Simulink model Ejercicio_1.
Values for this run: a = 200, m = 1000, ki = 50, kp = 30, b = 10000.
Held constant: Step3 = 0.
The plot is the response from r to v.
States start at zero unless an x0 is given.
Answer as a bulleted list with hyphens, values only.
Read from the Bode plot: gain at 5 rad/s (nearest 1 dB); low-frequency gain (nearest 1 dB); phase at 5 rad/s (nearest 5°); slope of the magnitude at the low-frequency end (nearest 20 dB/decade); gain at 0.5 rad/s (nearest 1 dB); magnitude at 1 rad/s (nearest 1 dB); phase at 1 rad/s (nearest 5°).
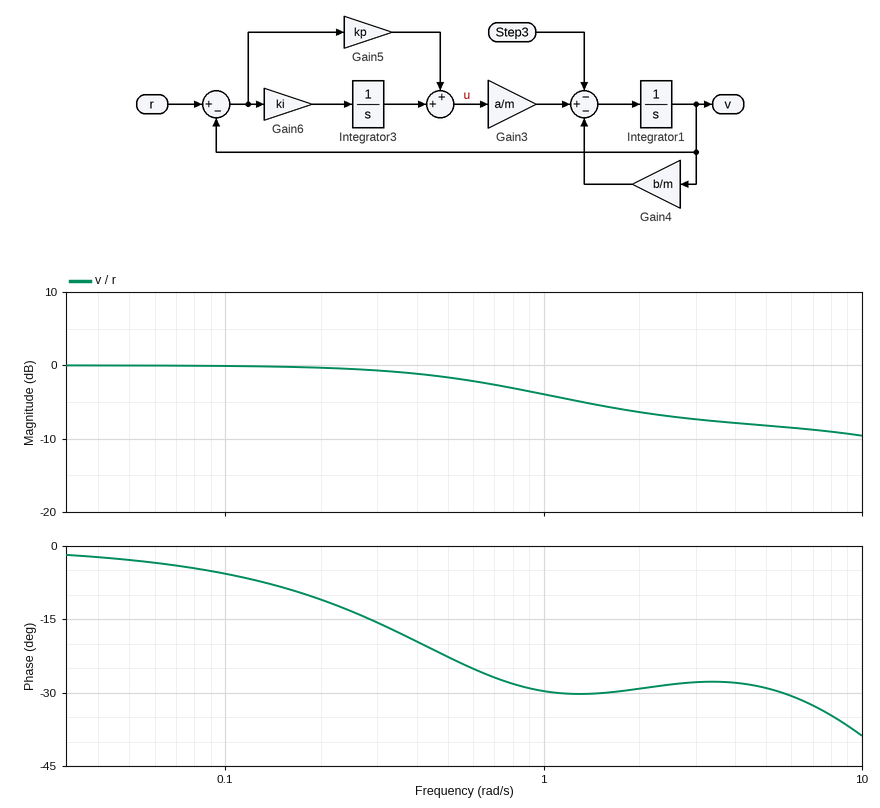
- -8 dB
- 0 dB
- -30°
- 0 dB/decade
- -2 dB
- -4 dB
- -30°
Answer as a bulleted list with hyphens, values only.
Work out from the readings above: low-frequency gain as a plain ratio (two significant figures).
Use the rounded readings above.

- 1.0
